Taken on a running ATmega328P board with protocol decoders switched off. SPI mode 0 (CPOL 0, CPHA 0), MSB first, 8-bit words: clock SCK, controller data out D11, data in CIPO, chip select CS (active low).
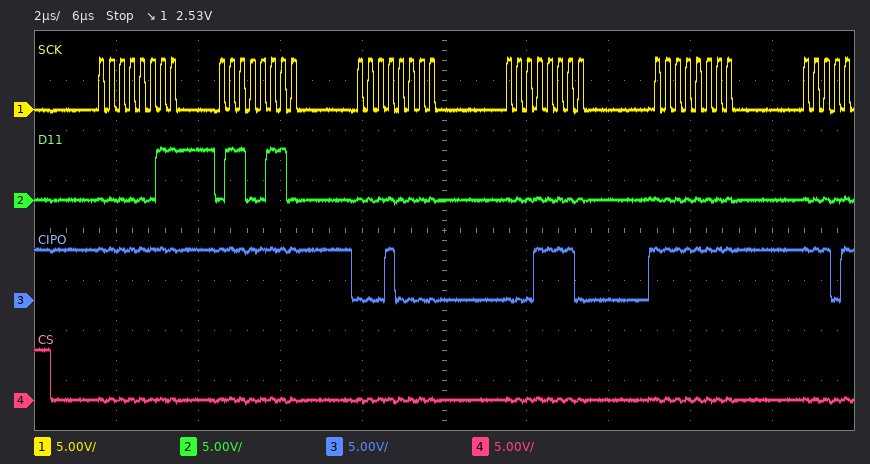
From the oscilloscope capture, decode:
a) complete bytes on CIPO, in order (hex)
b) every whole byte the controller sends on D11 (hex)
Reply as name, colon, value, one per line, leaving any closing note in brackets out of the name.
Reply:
complete bytes on CIPO, in order: FF FF 10 1E FF
every whole byte the controller sends on D11: 03 66 00 00 00
